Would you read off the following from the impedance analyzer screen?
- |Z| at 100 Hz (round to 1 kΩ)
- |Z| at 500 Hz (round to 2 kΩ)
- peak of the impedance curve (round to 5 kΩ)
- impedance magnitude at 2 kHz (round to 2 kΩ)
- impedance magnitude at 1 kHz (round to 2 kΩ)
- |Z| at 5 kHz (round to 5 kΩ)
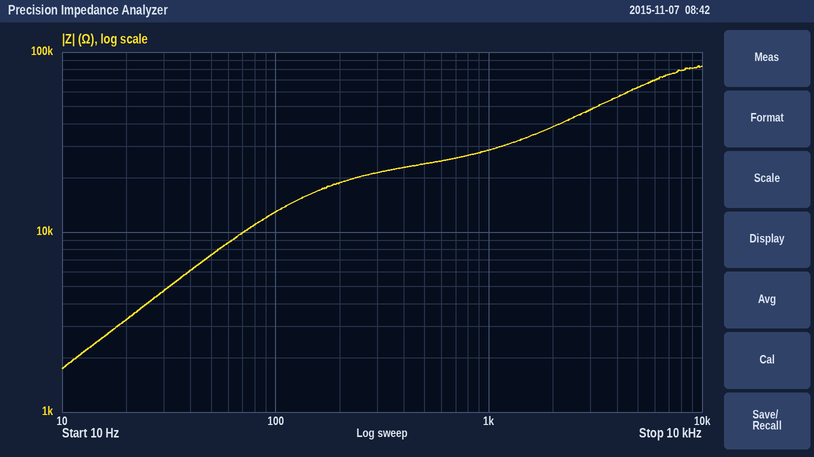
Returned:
13 kΩ
24 kΩ
85 kΩ
38 kΩ
28 kΩ
65 kΩ
